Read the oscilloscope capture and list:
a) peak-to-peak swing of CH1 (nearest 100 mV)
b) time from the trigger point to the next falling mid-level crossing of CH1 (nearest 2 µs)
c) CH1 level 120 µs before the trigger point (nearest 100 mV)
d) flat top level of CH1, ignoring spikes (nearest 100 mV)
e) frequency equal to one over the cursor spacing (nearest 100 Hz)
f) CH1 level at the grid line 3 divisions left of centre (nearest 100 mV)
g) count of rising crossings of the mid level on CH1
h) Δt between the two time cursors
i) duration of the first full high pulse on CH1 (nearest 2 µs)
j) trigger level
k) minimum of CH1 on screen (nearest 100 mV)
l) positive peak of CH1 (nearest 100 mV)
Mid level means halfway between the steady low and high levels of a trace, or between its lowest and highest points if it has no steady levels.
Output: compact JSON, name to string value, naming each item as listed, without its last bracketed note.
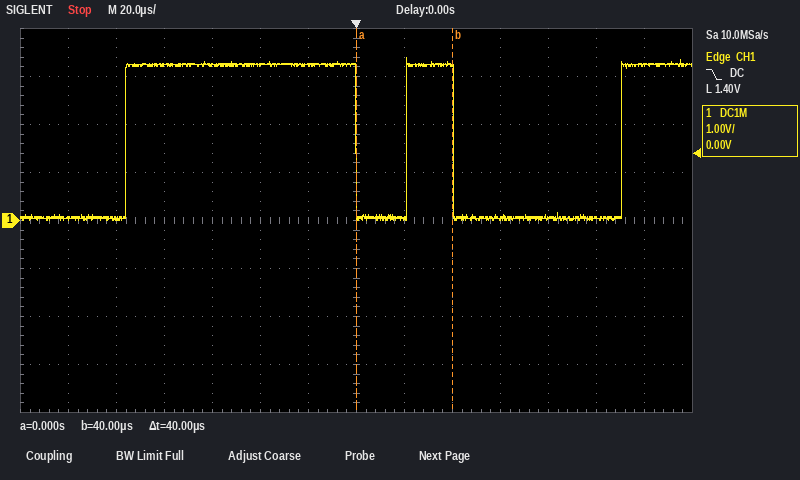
{"peak-to-peak swing of CH1": "3.4 V", "time from the trigger point to the next falling mid-level crossing of CH1": "40 µs", "CH1 level 120 µs before the trigger point": "0.0 V", "flat top level of CH1, ignoring spikes": "3.2 V", "frequency equal to one over the cursor spacing": "25.0 kHz", "CH1 level at the grid line 3 divisions left of centre": "3.2 V", "count of rising crossings of the mid level on CH1": "3", "Δt between the two time cursors": "40 µs", "duration of the first full high pulse on CH1": "96 µs", "trigger level": "1.40 V", "minimum of CH1 on screen": "0.0 V", "positive peak of CH1": "3.4 V"}
